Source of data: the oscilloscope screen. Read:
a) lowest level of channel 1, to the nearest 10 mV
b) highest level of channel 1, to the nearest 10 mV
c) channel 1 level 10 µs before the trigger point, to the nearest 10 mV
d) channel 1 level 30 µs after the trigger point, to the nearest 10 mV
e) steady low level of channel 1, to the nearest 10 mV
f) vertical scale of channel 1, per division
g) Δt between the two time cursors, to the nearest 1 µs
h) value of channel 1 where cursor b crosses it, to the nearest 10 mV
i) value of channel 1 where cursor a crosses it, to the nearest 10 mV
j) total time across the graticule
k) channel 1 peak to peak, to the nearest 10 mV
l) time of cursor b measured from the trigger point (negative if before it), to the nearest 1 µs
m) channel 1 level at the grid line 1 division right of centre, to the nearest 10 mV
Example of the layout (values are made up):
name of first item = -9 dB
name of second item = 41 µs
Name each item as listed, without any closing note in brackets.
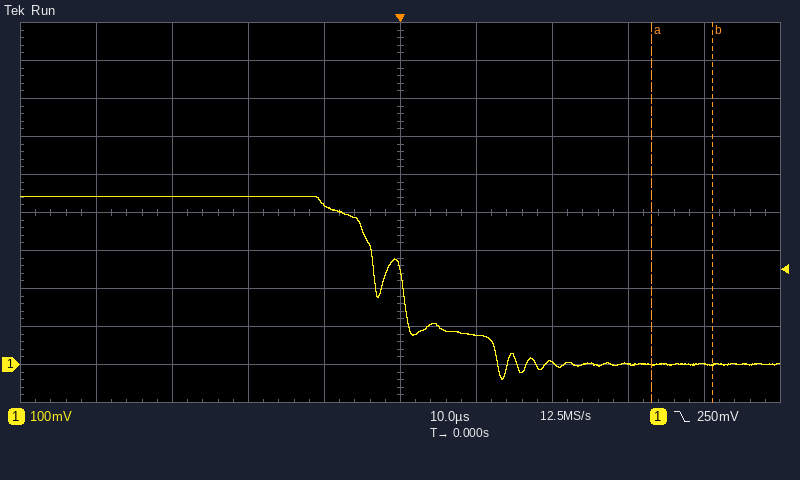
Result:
lowest level of channel 1, to the nearest 10 mV = -40 mV
highest level of channel 1, to the nearest 10 mV = 440 mV
channel 1 level 10 µs before the trigger point, to the nearest 10 mV = 420 mV
channel 1 level 30 µs after the trigger point, to the nearest 10 mV = 0 mV
steady low level of channel 1, to the nearest 10 mV = 0 mV
vertical scale of channel 1, per division = 100 mV
Δt between the two time cursors, to the nearest 1 µs = 8 µs
value of channel 1 where cursor b crosses it, to the nearest 10 mV = 0 mV
value of channel 1 where cursor a crosses it, to the nearest 10 mV = 0 mV
total time across the graticule = 100 µs
channel 1 peak to peak, to the nearest 10 mV = 480 mV
time of cursor b measured from the trigger point (negative if before it), to the nearest 1 µs = +41 µs
channel 1 level at the grid line 1 division right of centre, to the nearest 10 mV = 80 mV
